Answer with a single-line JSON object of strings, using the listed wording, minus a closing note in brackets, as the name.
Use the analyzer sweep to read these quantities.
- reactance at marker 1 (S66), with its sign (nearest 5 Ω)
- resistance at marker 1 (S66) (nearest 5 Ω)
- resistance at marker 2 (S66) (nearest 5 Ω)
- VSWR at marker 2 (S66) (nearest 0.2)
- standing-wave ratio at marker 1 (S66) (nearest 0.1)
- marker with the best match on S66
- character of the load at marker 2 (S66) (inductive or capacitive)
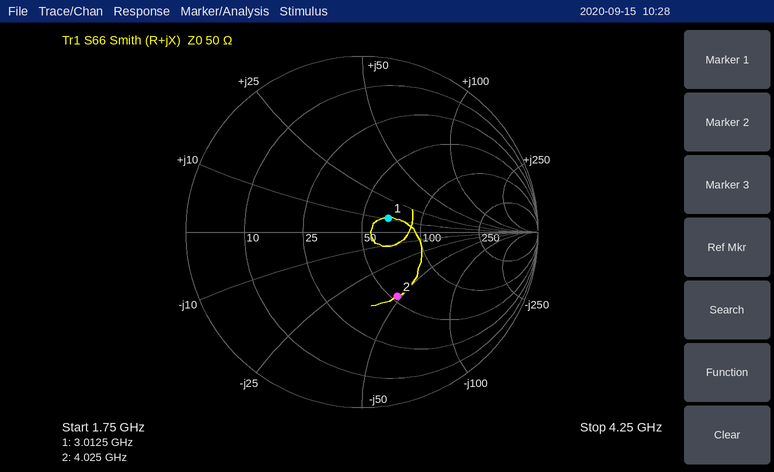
{"reactance at marker 1 (S66), with its sign": "+10 Ω", "resistance at marker 1 (S66)": "65 Ω", "resistance at marker 2 (S66)": "55 Ω", "VSWR at marker 2 (S66)": "2.4", "standing-wave ratio at marker 1 (S66)": "1.4", "marker with the best match on S66": "marker 1", "character of the load at marker 2 (S66)": "capacitive"}
